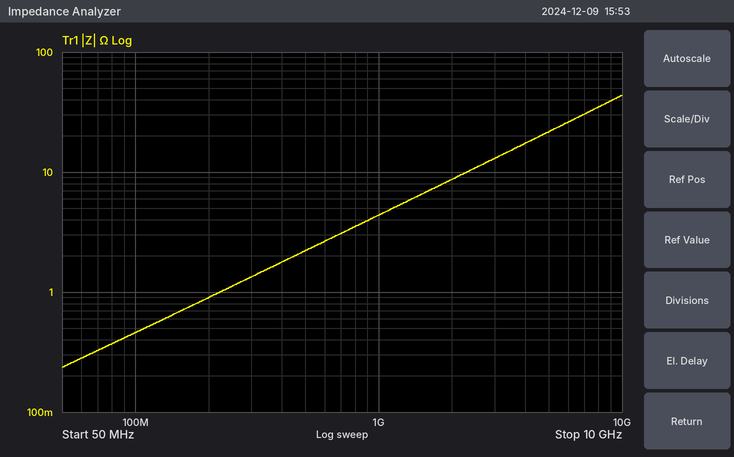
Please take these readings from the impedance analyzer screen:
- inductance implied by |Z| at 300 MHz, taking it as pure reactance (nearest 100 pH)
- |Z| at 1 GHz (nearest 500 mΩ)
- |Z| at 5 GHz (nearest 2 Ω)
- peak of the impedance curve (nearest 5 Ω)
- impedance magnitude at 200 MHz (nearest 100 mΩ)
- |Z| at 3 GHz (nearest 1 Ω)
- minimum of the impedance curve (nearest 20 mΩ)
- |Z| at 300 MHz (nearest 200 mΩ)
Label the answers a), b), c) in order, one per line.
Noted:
a) 700 pH
b) 4.5 Ω
c) 22 Ω
d) 45 Ω
e) 900 mΩ
f) 13 Ω
g) 240 mΩ
h) 1.4 Ω
